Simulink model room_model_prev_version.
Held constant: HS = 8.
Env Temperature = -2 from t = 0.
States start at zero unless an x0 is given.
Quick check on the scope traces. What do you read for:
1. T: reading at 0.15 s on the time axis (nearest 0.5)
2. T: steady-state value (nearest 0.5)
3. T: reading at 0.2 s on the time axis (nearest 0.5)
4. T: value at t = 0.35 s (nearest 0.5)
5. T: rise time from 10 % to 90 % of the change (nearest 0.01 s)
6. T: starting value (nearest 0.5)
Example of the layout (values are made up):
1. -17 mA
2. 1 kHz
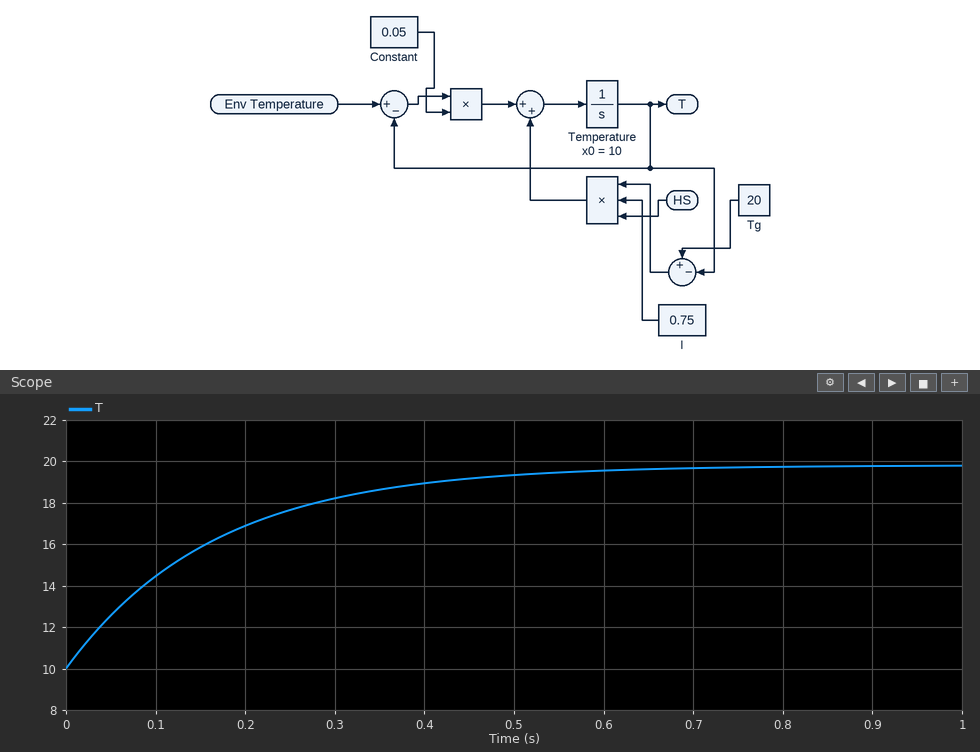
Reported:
1. 16.0
2. 20.0
3. 17.0
4. 18.5
5. 0.36 s
6. 10.0
